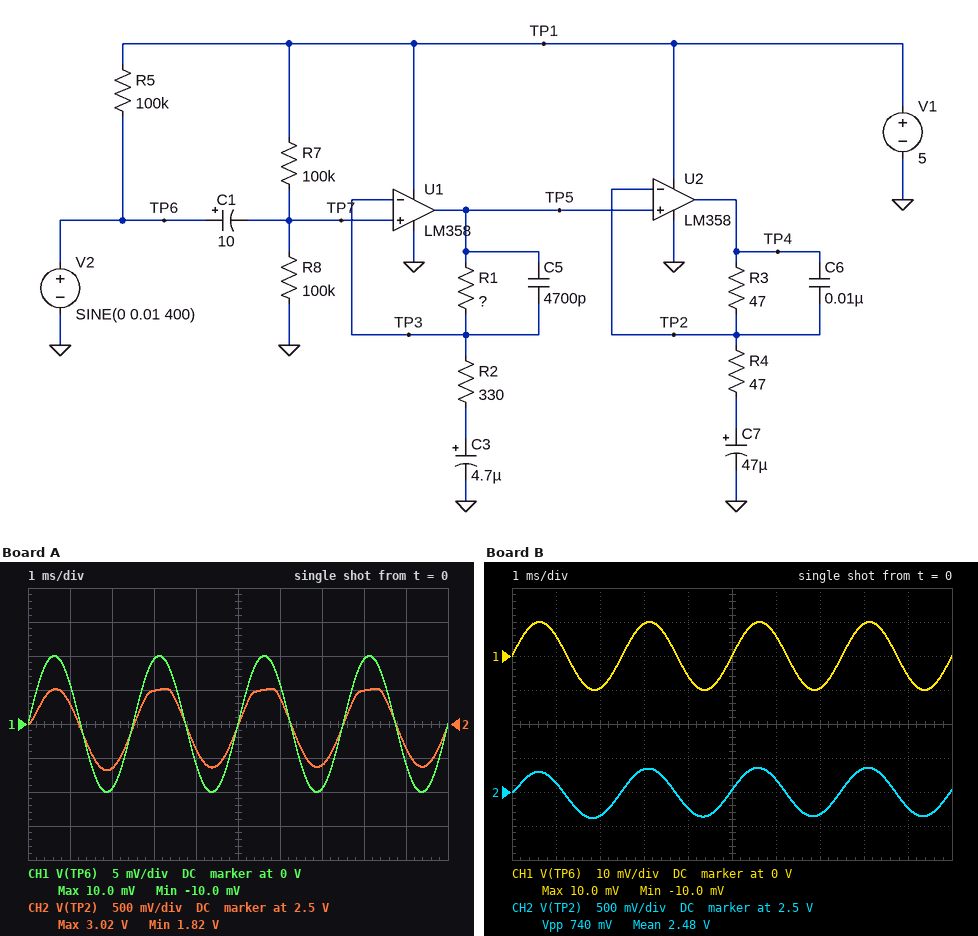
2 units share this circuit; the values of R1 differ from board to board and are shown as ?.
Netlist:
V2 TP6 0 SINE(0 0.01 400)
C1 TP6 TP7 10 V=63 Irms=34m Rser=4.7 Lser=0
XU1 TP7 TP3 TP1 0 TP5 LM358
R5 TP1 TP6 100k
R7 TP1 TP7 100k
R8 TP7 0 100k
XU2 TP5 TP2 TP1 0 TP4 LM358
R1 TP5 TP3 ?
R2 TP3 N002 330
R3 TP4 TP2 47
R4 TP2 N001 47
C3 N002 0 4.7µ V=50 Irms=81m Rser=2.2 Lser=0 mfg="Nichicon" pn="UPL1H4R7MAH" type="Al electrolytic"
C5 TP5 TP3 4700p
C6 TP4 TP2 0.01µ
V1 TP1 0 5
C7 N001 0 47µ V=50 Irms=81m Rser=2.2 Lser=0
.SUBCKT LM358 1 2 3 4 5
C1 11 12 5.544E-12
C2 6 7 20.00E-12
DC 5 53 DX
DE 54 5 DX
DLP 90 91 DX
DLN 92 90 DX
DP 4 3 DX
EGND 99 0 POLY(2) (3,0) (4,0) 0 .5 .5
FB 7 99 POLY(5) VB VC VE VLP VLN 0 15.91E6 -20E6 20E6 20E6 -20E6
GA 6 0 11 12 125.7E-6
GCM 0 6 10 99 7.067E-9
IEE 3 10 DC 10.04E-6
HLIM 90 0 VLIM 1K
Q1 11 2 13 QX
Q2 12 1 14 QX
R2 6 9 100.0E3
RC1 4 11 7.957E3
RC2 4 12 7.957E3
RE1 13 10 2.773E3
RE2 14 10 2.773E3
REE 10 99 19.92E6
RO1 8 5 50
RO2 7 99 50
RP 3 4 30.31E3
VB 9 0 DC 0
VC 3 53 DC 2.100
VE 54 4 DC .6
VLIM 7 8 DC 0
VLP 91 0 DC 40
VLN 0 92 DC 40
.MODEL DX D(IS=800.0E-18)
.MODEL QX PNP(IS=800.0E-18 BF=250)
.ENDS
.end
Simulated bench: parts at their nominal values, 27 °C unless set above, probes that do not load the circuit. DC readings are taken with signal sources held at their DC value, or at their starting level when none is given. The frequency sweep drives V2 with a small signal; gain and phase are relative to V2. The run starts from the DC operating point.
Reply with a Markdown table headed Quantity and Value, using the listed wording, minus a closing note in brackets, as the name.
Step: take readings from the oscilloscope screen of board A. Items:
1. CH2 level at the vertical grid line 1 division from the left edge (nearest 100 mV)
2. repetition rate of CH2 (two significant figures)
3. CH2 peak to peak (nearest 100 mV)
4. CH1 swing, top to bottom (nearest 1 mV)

| Quantity | Value |
|---|---|
| CH2 level at the vertical grid line 1 division from the left edge | 2.8 V |
| repetition rate of CH2 | 400 Hz |
| CH2 peak to peak | 1.2 V |
| CH1 swing, top to bottom | 20 mV |
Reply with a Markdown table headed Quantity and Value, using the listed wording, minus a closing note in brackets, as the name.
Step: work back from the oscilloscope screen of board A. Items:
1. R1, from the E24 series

| Quantity | Value |
|---|---|
| R1, from the E24 series | 22 kΩ |
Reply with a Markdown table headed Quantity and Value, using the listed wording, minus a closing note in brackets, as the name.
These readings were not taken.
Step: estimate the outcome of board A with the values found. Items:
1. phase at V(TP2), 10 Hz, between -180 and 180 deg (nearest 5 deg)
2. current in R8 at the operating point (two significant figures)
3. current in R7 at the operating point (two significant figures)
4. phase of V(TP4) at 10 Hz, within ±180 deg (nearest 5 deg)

| Quantity | Value |
|---|---|
| phase at V(TP2), 10 Hz, between -180 and 180 deg | 75 deg |
| current in R8 at the operating point | 25 µA |
| current in R7 at the operating point | 25 µA |
| phase of V(TP4) at 10 Hz, within ±180 deg | 85 deg |
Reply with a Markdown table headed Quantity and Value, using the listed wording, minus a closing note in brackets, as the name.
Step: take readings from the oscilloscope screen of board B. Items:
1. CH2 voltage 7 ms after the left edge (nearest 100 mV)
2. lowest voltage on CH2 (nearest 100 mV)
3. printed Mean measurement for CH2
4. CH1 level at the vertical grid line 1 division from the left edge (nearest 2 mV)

| Quantity | Value |
|---|---|
| CH2 voltage 7 ms after the left edge | 2.2 V |
| lowest voltage on CH2 | 2.1 V |
| printed Mean measurement for CH2 | 2.48 V |
| CH1 level at the vertical grid line 1 division from the left edge | 6 mV |
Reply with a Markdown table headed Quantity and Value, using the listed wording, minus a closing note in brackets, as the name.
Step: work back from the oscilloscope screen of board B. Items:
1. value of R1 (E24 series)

| Quantity | Value |
|---|---|
| value of R1 | 12 kΩ |
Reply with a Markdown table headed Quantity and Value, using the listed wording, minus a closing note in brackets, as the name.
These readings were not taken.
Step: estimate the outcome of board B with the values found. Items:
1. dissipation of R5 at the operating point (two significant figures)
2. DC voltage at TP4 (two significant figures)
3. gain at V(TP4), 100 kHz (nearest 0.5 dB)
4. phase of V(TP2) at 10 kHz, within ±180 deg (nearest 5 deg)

| Quantity | Value |
|---|---|
| dissipation of R5 at the operating point | 250 µW |
| DC voltage at TP4 | 2.5 V |
| gain at V(TP4), 100 kHz | 7.5 dB |
| phase of V(TP2) at 10 kHz, within ±180 deg | -70 deg |
